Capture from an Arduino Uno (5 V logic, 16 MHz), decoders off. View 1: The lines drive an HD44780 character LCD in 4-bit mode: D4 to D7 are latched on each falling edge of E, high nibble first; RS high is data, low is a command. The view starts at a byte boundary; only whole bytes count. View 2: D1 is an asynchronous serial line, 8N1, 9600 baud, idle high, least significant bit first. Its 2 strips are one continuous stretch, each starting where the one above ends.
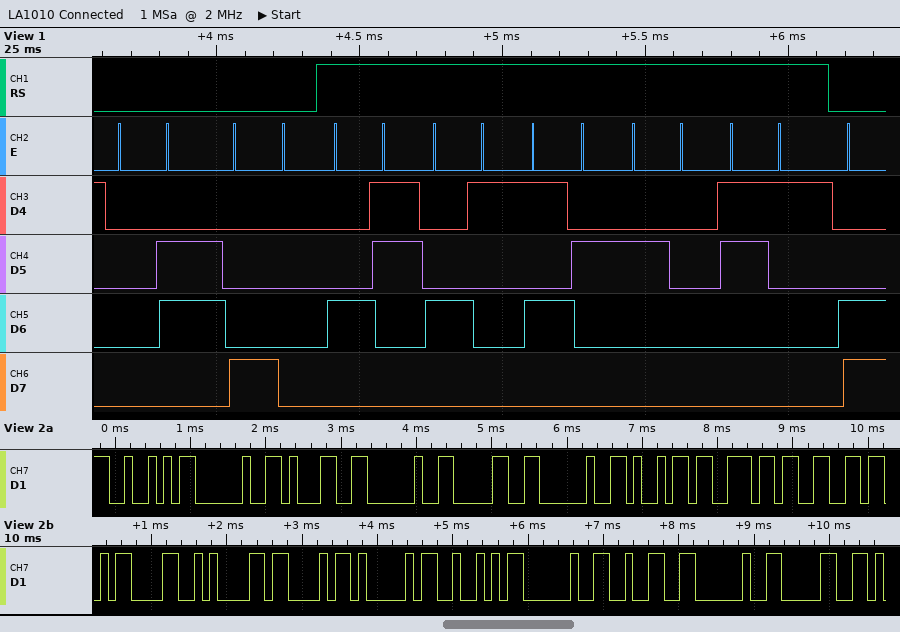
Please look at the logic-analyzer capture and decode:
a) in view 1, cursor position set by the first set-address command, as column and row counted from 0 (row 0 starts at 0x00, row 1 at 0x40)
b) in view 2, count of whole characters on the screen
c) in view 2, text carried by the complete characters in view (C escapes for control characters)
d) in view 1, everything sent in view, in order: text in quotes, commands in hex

column 0, row 0
18
"R 1 0 inf\r\nCAR 2 0"
0x06 0x80 "CAR 1"
